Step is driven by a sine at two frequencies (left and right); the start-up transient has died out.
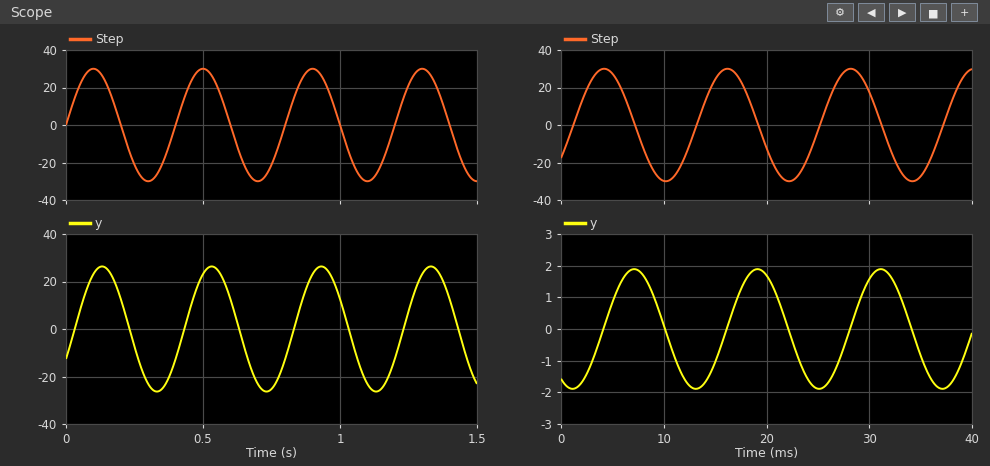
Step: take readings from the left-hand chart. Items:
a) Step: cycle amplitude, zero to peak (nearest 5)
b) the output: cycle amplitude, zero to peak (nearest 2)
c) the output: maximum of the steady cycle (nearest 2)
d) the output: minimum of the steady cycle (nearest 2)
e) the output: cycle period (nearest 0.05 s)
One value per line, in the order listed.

30
26
26
-26
0.40 s
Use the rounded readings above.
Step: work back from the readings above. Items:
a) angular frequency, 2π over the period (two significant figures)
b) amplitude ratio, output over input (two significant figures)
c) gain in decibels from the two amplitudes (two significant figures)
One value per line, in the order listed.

16 rad/s
0.87
-1.2 dB
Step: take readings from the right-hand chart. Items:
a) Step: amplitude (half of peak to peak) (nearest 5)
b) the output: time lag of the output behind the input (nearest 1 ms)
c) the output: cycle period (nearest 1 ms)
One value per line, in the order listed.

30
3 ms
12 ms
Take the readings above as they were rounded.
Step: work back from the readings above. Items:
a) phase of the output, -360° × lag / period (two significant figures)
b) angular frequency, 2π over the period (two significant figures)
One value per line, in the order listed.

-90°
0.52 rad/ms
